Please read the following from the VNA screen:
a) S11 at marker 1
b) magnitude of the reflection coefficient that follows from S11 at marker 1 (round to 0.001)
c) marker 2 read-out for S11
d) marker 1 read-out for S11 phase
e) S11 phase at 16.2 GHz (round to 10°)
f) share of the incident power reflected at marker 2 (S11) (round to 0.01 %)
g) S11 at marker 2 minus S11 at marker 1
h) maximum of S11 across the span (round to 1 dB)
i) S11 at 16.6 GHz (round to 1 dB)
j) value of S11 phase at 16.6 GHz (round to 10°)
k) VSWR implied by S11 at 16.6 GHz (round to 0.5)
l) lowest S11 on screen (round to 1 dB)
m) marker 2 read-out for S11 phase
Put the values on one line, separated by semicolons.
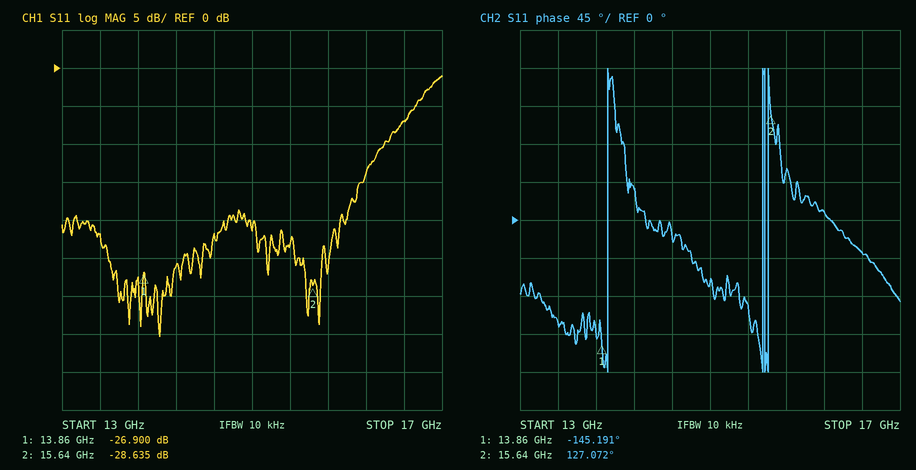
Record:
-26.900 dB; 0.045; -28.635 dB; -145.191°; 10°; 0.14 %; -1.735 dB; -1 dB; -7 dB; -40°; 2.5; -35 dB; 127.072°
